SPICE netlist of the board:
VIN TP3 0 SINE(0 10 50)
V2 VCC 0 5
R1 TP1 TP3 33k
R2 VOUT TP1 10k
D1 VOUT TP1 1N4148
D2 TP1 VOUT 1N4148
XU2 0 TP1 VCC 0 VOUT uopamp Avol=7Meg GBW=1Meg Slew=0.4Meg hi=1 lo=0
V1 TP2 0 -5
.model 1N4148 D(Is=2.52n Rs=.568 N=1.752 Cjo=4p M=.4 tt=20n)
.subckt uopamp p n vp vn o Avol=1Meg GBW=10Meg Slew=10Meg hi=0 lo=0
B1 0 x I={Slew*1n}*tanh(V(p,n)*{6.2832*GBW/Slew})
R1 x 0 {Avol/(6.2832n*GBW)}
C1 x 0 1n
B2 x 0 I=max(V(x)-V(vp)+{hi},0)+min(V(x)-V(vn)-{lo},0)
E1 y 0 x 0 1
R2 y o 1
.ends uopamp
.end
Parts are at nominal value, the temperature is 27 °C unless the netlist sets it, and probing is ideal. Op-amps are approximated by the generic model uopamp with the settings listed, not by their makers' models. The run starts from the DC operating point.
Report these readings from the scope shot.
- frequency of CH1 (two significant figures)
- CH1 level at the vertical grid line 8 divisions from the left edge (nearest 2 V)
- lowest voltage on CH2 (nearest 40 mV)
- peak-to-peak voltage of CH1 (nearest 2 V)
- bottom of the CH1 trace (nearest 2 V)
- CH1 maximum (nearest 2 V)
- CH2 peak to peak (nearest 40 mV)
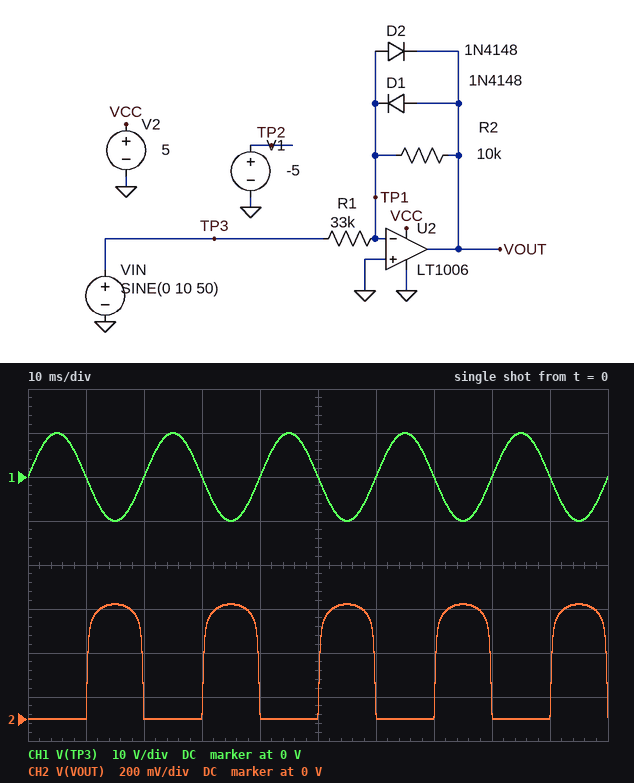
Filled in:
50 Hz
0 V
0 V
20 V
-10 V
10 V
520 mV
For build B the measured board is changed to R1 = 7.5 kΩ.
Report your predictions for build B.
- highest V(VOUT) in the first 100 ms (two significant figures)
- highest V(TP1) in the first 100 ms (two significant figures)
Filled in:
600 mV
590 mV
